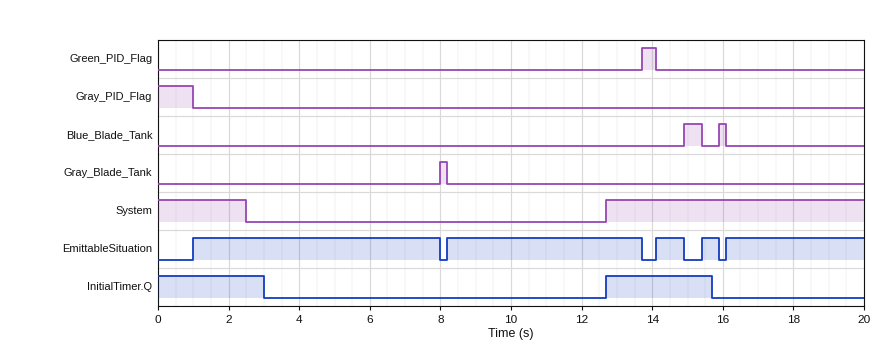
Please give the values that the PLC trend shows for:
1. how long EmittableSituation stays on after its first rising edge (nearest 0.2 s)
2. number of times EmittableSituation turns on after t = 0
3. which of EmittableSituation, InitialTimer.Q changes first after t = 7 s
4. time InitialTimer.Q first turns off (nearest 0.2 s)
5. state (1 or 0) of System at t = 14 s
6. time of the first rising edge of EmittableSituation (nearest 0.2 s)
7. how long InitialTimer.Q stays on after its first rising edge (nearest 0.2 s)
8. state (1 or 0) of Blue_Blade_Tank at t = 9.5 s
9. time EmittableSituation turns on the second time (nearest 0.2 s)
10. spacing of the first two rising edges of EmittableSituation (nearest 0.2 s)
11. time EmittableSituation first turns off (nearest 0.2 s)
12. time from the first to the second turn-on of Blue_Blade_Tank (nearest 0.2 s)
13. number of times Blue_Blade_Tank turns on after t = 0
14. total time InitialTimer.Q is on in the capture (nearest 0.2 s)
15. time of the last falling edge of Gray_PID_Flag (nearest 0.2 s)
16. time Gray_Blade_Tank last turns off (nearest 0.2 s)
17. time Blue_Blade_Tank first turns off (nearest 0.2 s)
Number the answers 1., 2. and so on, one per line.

1. 7.0 s
2. 5
3. EmittableSituation
4. 3.0 s
5. 1
6. 1.0 s
7. 3.0 s
8. 0
9. 8.2 s
10. 7.2 s
11. 8.0 s
12. 1.0 s
13. 2
14. 6.0 s
15. 1.0 s
16. 8.2 s
17. 15.4 s
